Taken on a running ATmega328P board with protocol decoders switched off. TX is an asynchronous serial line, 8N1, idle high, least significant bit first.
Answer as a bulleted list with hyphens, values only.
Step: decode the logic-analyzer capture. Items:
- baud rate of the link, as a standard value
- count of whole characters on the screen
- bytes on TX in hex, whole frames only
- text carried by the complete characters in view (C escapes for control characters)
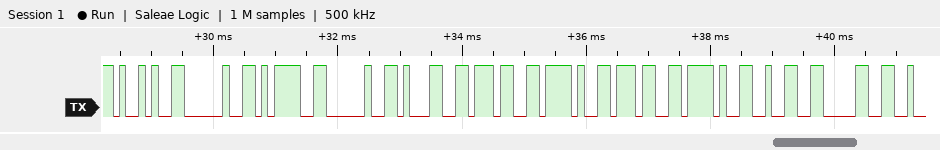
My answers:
- 9600 baud
- 11
- 0x29 0x20 0x3D 0x20 0x31 0x37 0x2F 0x37 0x2F 0x32 0x30
- ") = 17/7/20"
